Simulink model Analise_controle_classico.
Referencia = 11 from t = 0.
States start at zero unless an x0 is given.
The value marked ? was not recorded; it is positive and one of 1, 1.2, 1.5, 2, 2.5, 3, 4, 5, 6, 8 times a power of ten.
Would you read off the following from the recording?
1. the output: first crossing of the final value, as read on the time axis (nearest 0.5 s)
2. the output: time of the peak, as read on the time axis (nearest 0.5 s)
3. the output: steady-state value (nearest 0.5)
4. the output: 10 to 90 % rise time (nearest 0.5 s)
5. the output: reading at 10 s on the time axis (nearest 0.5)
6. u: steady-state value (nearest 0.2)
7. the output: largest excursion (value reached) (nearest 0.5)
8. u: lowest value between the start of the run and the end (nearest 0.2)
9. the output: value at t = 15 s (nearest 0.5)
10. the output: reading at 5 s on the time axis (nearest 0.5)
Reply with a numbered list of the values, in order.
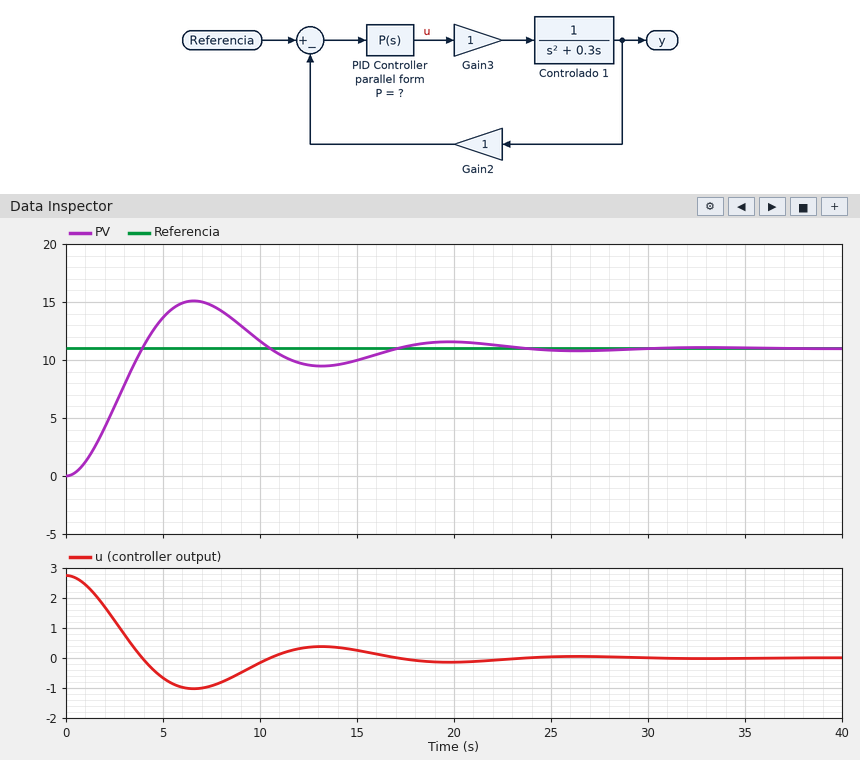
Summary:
1. 4.0 s
2. 6.5 s
3. 11.0
4. 2.5 s
5. 11.5
6. 0.0
7. 15.0
8. -1.0
9. 10.0
10. 13.5
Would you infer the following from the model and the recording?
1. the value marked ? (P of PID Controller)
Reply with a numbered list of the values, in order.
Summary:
1. 0.25
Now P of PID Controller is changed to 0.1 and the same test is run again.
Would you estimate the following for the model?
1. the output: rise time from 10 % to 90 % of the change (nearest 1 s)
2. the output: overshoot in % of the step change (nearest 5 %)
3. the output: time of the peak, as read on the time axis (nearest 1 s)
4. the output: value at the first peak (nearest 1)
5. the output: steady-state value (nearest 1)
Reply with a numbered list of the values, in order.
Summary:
1. 5 s
2. 20 %
3. 11 s
4. 13
5. 11
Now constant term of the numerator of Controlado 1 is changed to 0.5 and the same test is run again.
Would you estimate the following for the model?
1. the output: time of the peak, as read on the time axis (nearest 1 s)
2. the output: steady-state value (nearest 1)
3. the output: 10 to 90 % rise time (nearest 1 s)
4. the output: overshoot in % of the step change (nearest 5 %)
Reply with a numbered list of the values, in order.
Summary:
1. 10 s
2. 11
3. 4 s
4. 25 %
